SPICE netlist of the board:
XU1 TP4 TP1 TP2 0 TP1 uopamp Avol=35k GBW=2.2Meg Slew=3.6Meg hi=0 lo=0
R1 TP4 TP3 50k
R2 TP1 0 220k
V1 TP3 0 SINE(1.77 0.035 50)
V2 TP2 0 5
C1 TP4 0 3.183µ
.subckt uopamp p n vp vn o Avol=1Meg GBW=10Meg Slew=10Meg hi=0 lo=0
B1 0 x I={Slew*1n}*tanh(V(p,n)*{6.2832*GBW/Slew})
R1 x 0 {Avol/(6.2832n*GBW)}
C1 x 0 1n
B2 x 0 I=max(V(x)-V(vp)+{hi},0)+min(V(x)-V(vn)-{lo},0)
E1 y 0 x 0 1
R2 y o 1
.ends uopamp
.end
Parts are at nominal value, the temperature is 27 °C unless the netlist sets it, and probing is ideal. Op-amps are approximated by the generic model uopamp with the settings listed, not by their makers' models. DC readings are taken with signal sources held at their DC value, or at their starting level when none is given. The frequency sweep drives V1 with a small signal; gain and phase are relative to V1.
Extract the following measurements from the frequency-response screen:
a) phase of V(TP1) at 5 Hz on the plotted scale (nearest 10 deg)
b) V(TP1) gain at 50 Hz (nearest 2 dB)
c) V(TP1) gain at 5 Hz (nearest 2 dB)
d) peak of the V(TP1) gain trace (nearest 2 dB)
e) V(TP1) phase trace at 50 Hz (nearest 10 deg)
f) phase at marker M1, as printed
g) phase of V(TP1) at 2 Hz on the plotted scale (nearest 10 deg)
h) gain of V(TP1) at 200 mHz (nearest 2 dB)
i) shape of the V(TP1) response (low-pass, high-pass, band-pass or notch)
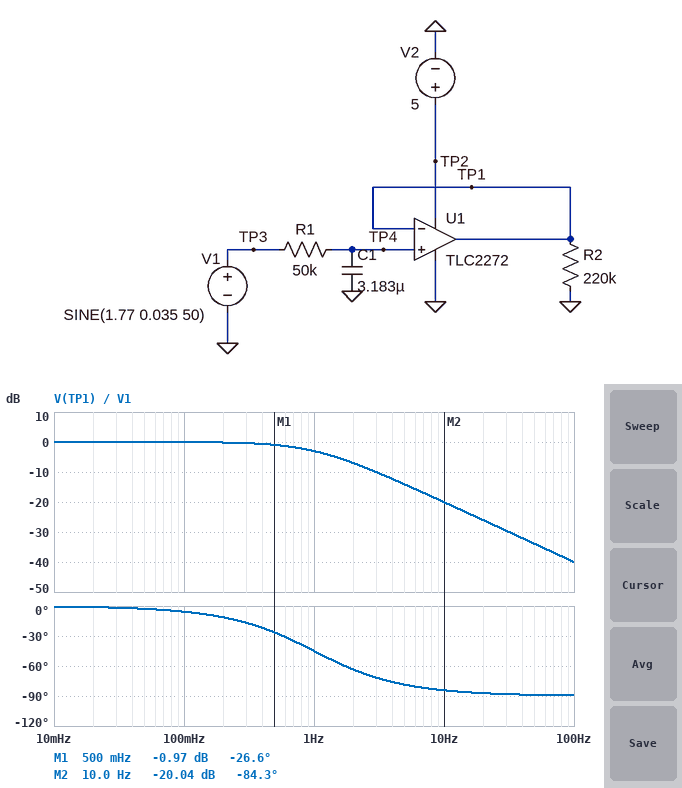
-80 deg
-34 dB
-14 dB
0 dB
-90 deg
-26.6 deg
-60 deg
0 dB
low-pass
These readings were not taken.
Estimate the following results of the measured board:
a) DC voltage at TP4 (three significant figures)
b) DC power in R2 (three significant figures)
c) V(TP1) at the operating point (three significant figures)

1.77 V
14.2 µW
1.77 V
